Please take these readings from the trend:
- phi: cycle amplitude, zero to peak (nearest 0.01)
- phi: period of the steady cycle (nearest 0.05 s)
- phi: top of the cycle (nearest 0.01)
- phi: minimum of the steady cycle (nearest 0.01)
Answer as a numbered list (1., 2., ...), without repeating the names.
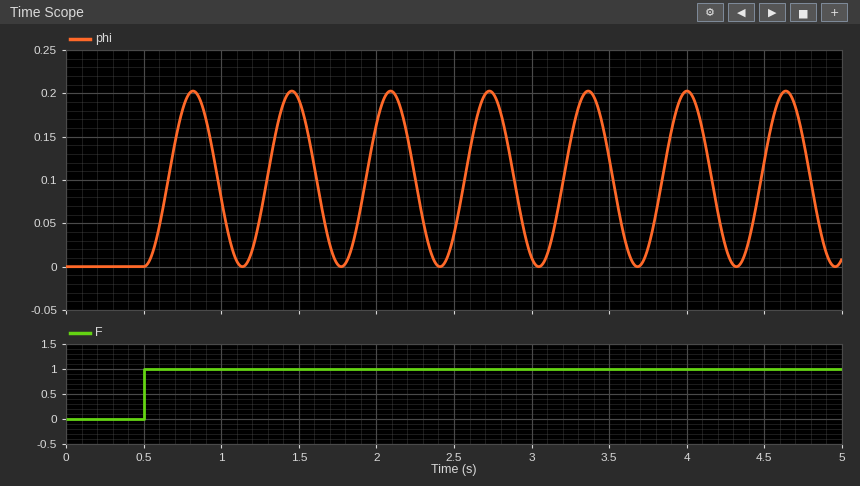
1. 0.10
2. 0.65 s
3. 0.20
4. 0.00
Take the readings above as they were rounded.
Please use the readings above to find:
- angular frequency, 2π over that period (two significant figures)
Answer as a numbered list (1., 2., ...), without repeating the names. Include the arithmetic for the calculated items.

1. 2π / 0.65 = 9.7 rad/s
